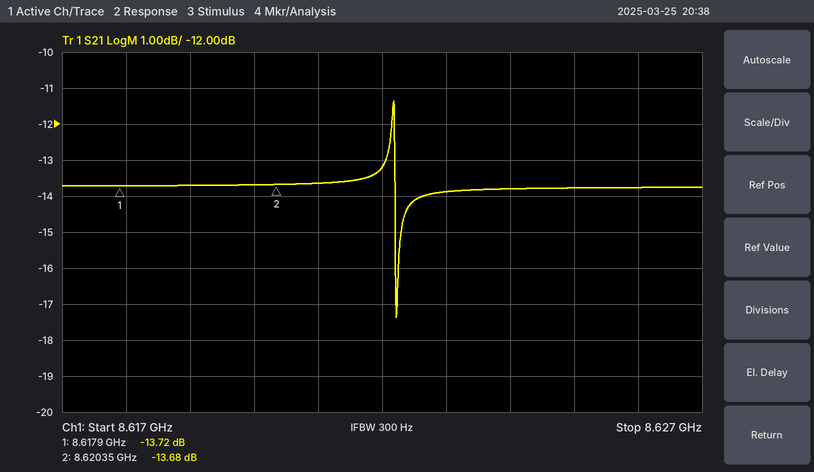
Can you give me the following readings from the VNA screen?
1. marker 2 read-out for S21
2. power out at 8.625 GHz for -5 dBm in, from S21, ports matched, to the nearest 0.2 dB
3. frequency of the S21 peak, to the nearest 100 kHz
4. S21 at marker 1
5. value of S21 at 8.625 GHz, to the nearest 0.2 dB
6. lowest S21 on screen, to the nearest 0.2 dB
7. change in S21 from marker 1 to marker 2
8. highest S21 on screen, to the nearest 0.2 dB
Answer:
-13.68 dB
-18.8 dBm
8.6222 GHz
-13.72 dB
-13.8 dB
-17.4 dB
0.04 dB
-11.4 dB
